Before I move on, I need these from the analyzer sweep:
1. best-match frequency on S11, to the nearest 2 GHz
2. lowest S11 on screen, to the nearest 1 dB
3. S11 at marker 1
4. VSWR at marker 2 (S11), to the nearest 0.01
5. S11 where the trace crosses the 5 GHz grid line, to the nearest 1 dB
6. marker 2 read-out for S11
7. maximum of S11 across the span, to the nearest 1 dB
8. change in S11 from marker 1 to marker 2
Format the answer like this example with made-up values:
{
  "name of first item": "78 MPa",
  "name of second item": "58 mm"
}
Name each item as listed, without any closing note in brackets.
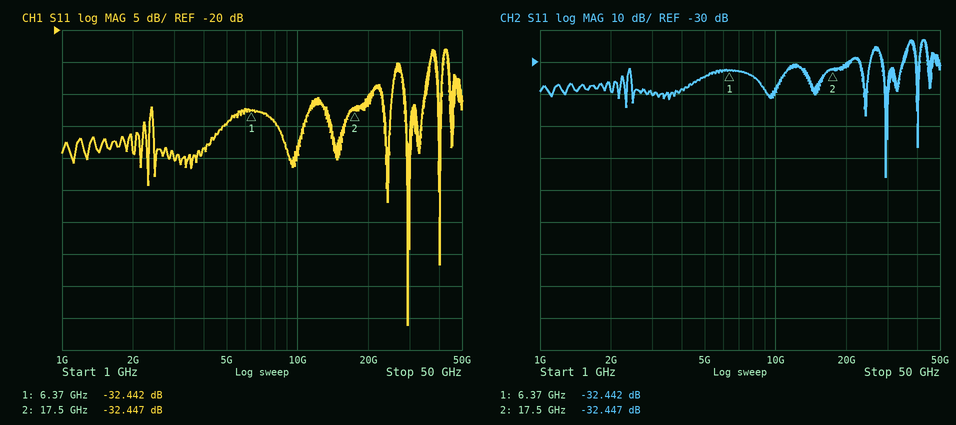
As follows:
{
  "best-match frequency on S11, to the nearest 2 GHz": "30 GHz",
  "lowest S11 on screen, to the nearest 1 dB": "-66 dB",
  "S11 at marker 1": "-32.442 dB",
  "VSWR at marker 2 (S11), to the nearest 0.01": "1.05",
  "S11 where the trace crosses the 5 GHz grid line, to the nearest 1 dB": "-35 dB",
  "marker 2 read-out for S11": "-32.447 dB",
  "maximum of S11 across the span, to the nearest 1 dB": "-23 dB",
  "change in S11 from marker 1 to marker 2": "-0.005 dB"
}
